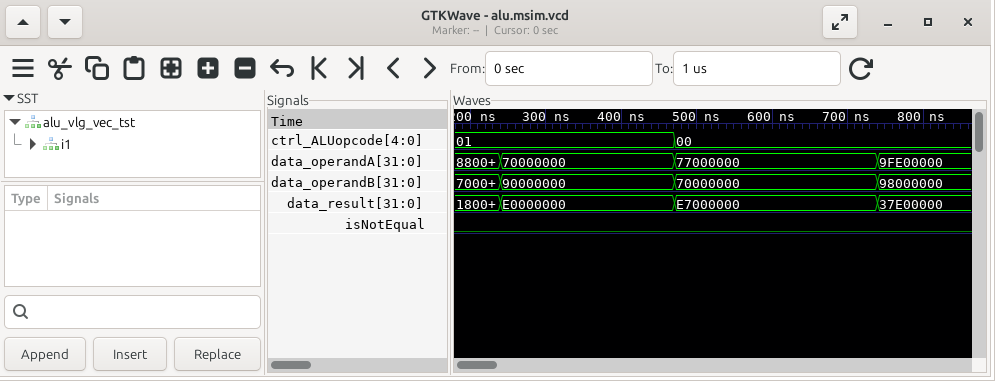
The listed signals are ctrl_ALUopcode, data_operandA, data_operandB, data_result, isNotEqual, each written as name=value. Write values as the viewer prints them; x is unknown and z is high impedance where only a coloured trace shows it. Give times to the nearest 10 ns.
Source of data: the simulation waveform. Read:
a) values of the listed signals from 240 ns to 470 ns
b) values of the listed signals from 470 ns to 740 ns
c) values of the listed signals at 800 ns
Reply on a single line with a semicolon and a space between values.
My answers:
ctrl_ALUopcode=01, data_operandA=70000000, data_operandB=90000000, data_result=E0000000, isNotEqual=0; ctrl_ALUopcode=00, data_operandA=77000000, data_operandB=70000000, data_result=E7000000, isNotEqual=0; ctrl_ALUopcode=00, data_operandA=9FE00000, data_operandB=98000000, data_result=37E00000, isNotEqual=0
